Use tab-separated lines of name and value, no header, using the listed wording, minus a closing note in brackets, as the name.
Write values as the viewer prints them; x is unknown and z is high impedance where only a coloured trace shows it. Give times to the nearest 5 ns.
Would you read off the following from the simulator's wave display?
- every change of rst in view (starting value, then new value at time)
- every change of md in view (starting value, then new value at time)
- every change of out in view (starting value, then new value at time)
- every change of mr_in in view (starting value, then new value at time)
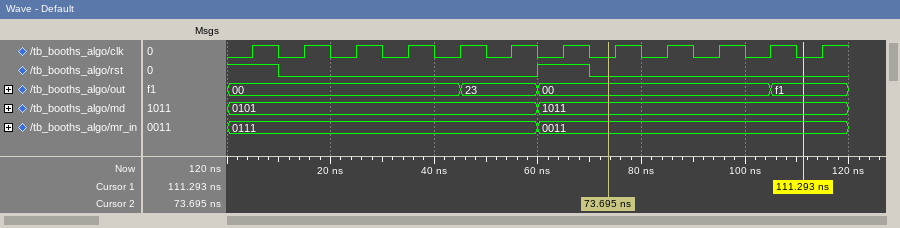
every change of rst in view	1, 0 at 10 ns, 1 at 60 ns, 0 at 70 ns
every change of md in view	0101, 1011 at 60 ns
every change of out in view	00, 23 at 45 ns, 00 at 60 ns, f1 at 105 ns
every change of mr_in in view	0111, 0011 at 60 ns
